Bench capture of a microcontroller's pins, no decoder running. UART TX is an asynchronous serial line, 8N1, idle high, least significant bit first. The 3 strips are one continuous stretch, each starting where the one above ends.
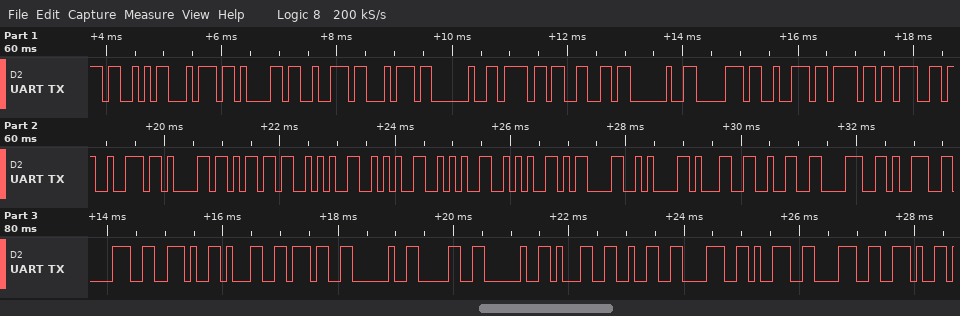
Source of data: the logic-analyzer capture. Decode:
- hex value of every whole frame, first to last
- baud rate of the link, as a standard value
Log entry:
53 74 61 72 74 20 6F 66 20 70 72 6F 67 72 61 6D 2A 2A 2A 2A 0D 0A 31 32 38 39 38 2E 31 37 20 30 20 31 32 38 39 38 2E
9600 baud
